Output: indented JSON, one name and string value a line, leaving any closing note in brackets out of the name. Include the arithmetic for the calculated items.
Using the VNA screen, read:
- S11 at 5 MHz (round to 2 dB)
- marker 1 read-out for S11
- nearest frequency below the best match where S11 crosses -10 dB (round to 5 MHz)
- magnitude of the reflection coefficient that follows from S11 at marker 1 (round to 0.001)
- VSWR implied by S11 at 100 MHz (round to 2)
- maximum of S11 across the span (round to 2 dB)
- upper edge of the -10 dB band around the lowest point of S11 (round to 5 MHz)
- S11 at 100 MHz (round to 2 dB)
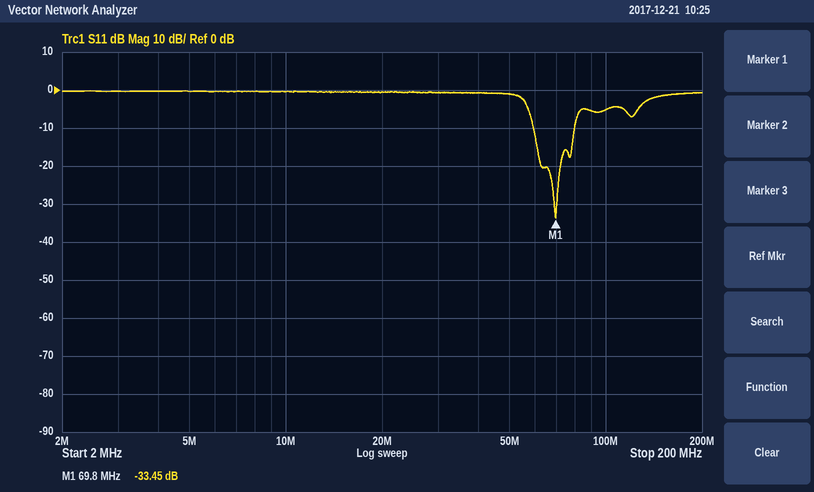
{
  "S11 at 5 MHz": "0 dB",
  "marker 1 read-out for S11": "-33.45 dB",
  "nearest frequency below the best match where S11 crosses -10 dB": "60 MHz",
  "magnitude of the reflection coefficient that follows from S11 at marker 1": "10^(-33.45/20) ≈ 0.021",
  "VSWR implied by S11 at 100 MHz": "|Γ| = 10^(-6/20) = 0.5012; VSWR = (1 + 0.5012)/(1 − 0.5012) ≈ 3.01, so 4 to the nearest 2",
  "maximum of S11 across the span": "0 dB",
  "upper edge of the -10 dB band around the lowest point of S11": "80 MHz",
  "S11 at 100 MHz": "-6 dB"
}
